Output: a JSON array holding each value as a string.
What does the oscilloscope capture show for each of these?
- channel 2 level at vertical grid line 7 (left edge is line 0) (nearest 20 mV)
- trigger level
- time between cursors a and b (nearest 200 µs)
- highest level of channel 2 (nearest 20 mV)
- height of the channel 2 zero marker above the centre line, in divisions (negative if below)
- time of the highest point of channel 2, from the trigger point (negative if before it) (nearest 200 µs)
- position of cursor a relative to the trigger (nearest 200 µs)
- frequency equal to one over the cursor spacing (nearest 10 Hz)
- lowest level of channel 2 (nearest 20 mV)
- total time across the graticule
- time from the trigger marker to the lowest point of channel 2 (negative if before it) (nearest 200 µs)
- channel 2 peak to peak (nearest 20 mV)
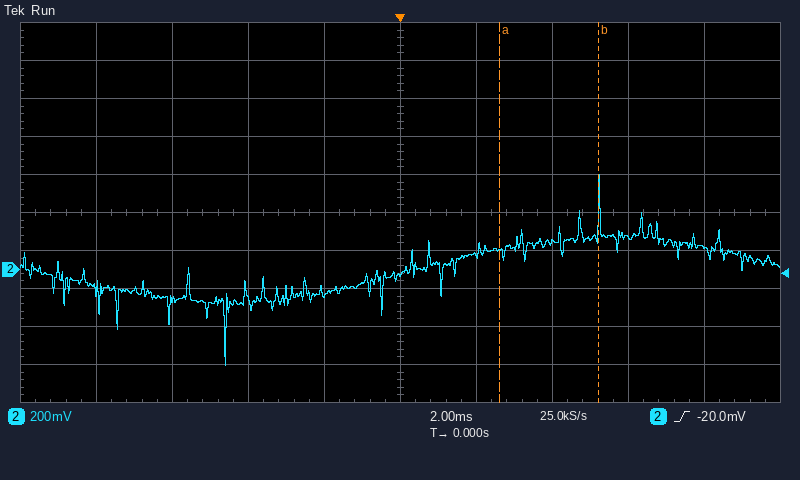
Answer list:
["140 mV", "-20.0 mV", "2.6 ms", "500 mV", "-1.5 div", "+5.2 ms", "+2.6 ms", "380 Hz", "-500 mV", "20 ms", "-4.6 ms", "1.00 V"]
